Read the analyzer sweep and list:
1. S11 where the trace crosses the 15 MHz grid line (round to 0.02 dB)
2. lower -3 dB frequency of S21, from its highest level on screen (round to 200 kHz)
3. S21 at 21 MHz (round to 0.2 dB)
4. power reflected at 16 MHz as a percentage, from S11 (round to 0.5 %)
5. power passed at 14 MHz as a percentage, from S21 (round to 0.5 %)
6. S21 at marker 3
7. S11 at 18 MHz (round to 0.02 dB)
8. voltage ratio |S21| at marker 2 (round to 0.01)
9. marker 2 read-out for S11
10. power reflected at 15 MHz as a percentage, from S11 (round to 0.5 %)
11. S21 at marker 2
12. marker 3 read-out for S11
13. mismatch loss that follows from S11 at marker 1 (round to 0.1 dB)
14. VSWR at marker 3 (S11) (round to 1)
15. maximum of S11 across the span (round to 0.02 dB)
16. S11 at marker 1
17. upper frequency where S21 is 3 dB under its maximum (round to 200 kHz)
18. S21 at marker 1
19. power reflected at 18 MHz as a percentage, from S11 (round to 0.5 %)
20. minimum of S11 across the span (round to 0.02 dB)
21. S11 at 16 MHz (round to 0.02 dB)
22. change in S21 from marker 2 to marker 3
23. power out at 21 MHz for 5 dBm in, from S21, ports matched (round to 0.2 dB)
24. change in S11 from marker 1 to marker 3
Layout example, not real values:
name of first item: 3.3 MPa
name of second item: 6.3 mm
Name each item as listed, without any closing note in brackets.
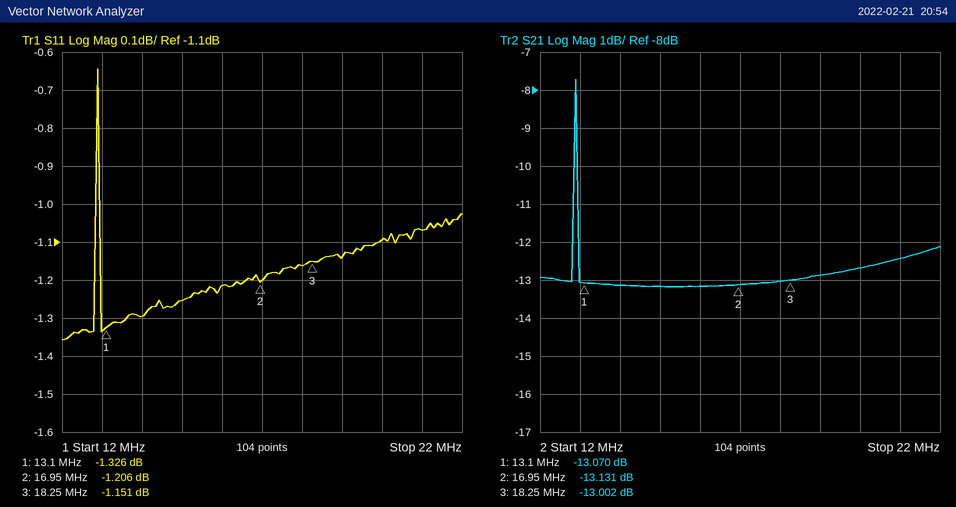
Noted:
S11 where the trace crosses the 15 MHz grid line: -1.26 dB
lower -3 dB frequency of S21, from its highest level on screen: 12.8 MHz
S21 at 21 MHz: -12.4 dB
power reflected at 16 MHz as a percentage, from S11: 75.5 %
power passed at 14 MHz as a percentage, from S21: 5.0 %
S21 at marker 3: -13.002 dB
S11 at 18 MHz: -1.16 dB
voltage ratio |S21| at marker 2: 0.22
marker 2 read-out for S11: -1.206 dB
power reflected at 15 MHz as a percentage, from S11: 75.0 %
S21 at marker 2: -13.131 dB
marker 3 read-out for S11: -1.151 dB
mismatch loss that follows from S11 at marker 1: 5.8 dB
VSWR at marker 3 (S11): 15
maximum of S11 across the span: -0.64 dB
S11 at marker 1: -1.326 dB
upper frequency where S21 is 3 dB under its maximum: 13.0 MHz
S21 at marker 1: -13.070 dB
power reflected at 18 MHz as a percentage, from S11: 76.5 %
minimum of S11 across the span: -1.36 dB
S11 at 16 MHz: -1.22 dB
change in S21 from marker 2 to marker 3: 0.129 dB
power out at 21 MHz for 5 dBm in, from S21, ports matched: -7.4 dBm
change in S11 from marker 1 to marker 3: 0.175 dB
